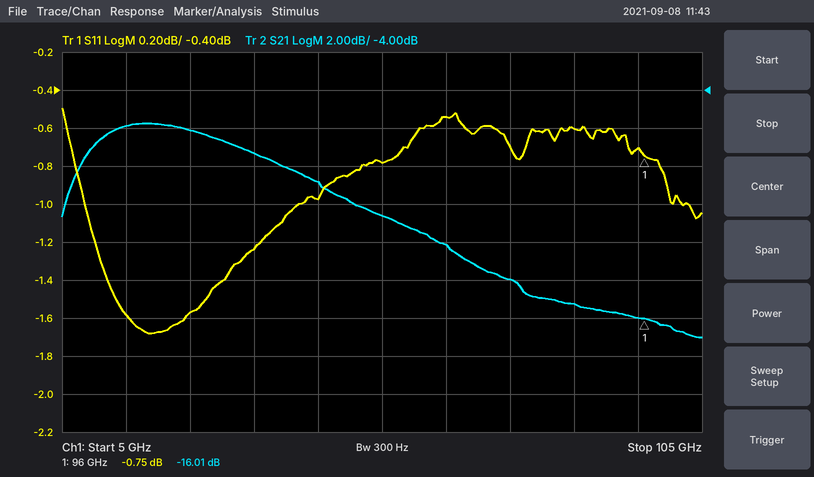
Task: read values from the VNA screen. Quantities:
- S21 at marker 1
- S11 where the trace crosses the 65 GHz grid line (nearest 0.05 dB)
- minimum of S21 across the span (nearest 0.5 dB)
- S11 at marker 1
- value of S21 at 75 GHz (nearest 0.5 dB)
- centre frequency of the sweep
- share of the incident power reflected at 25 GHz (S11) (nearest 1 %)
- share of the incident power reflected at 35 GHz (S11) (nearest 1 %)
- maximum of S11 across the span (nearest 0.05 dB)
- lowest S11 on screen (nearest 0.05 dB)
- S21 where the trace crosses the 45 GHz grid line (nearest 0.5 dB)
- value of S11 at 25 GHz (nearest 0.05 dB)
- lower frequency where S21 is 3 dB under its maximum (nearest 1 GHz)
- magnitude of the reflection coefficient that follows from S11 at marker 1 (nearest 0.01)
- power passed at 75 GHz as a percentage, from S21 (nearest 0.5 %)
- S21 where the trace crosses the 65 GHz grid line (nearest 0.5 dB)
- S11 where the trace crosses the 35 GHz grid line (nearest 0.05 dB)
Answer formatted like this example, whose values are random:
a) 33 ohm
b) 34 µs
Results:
a) -16.01 dB
b) -0.55 dB
c) -17.0 dB
d) -0.75 dB
e) -14.0 dB
f) 55 GHz
g) 70 %
h) 75 %
i) -0.50 dB
j) -1.70 dB
k) -9.0 dB
l) -1.55 dB
m) 7 GHz
n) 0.92
o) 4.0 %
p) -12.0 dB
q) -1.25 dB
